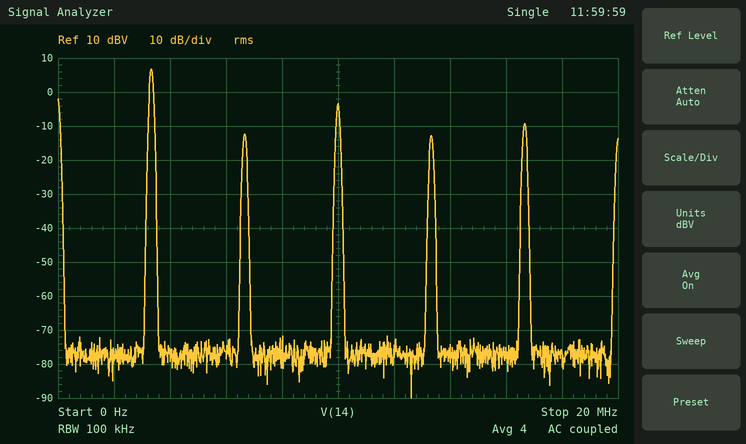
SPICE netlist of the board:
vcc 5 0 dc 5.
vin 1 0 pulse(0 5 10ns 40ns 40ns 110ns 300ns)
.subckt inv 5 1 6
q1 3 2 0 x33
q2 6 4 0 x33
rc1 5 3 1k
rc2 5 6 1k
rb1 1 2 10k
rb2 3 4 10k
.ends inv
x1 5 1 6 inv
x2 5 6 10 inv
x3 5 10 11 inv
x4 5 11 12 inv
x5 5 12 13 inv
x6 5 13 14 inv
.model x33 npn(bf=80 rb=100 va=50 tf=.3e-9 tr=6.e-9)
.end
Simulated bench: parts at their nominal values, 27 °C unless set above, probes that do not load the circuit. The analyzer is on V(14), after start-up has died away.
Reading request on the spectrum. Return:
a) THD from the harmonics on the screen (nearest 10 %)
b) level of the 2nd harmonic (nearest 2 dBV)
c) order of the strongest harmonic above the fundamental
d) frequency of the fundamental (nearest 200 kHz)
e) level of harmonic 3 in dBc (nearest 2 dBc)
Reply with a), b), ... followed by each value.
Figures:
a) 40 %
b) -12 dBV
c) 3
d) 3.4 MHz
e) -10 dBc
